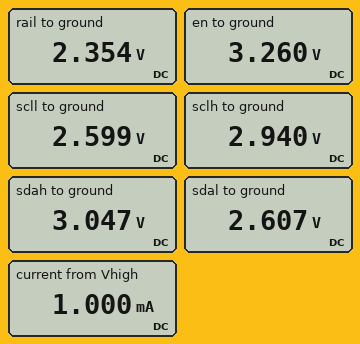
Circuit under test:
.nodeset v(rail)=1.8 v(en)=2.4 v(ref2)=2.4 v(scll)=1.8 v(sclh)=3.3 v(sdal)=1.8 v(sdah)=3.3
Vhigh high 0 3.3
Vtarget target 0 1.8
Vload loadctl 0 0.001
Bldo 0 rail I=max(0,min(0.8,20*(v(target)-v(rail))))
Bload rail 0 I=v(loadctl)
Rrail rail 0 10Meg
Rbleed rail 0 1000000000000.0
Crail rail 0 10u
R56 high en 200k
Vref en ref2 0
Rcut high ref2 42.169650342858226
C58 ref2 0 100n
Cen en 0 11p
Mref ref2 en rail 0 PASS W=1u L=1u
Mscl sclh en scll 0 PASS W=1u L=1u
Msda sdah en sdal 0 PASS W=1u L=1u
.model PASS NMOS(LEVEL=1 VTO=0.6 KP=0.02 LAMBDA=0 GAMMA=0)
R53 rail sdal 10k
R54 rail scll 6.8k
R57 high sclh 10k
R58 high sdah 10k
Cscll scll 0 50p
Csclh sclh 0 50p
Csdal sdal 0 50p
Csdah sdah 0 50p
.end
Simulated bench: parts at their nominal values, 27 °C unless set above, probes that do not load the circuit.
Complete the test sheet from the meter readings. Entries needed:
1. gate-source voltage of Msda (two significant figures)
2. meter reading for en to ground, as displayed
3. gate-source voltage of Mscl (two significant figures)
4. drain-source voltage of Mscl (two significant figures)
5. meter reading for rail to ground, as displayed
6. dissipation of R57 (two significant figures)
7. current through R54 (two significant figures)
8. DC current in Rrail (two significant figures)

650 mV
3.260 V
660 mV
340 mV
2.354 V
13 µW
36 µA
240 nA
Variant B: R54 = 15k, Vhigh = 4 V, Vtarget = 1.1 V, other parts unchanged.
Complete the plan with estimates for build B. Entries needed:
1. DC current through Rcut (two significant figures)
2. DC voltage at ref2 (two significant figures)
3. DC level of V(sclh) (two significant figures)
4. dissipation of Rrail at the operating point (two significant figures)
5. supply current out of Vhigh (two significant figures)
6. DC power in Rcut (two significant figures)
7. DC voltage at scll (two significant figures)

960 µA
4.0 V
3.8 V
930 nW
1.0 mA
39 µW
3.3 V
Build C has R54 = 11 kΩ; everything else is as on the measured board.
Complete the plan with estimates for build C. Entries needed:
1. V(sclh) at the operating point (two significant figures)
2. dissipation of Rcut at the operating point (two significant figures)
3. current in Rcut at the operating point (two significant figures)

3.1 V
38 µW
950 µA
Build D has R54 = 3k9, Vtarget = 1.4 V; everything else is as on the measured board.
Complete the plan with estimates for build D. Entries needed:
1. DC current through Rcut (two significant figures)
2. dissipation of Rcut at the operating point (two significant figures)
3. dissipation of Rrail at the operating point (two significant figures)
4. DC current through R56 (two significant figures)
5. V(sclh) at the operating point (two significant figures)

920 µA
35 µW
560 nW
190 nA
2.7 V
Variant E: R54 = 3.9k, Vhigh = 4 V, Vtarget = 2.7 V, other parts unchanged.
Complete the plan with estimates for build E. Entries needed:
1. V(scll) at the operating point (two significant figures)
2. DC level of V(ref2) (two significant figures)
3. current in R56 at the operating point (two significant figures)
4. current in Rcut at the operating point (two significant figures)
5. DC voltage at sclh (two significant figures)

3.3 V
4.0 V
190 nA
920 µA
3.4 V
